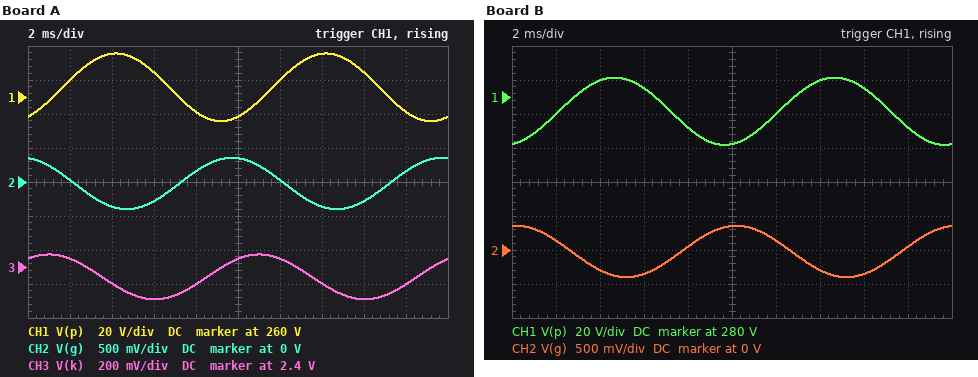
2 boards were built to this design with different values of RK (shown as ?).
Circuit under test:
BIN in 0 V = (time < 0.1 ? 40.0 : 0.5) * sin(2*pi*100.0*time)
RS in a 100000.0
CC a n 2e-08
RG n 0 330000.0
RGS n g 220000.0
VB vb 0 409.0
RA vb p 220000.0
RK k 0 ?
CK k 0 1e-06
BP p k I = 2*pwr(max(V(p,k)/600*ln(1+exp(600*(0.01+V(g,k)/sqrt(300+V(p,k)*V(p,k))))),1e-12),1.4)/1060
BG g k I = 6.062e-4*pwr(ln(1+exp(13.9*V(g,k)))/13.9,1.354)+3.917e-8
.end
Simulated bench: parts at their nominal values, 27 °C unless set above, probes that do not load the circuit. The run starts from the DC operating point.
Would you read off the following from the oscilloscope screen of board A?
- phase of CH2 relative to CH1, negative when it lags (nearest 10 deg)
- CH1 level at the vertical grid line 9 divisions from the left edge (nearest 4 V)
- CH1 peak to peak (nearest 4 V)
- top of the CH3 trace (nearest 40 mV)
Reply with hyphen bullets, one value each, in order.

- 160 deg
- 252 V
- 40 V
- 2.48 V
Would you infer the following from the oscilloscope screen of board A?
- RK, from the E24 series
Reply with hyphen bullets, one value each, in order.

- 3.6 kΩ
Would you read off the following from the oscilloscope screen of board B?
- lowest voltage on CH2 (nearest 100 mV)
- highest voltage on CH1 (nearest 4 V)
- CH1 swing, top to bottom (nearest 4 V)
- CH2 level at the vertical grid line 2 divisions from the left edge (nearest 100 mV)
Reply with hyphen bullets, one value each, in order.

- -400 mV
- 292 V
- 40 V
- -300 mV
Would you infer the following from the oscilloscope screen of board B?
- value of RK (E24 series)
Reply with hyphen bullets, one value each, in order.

- 3.9 kΩ
